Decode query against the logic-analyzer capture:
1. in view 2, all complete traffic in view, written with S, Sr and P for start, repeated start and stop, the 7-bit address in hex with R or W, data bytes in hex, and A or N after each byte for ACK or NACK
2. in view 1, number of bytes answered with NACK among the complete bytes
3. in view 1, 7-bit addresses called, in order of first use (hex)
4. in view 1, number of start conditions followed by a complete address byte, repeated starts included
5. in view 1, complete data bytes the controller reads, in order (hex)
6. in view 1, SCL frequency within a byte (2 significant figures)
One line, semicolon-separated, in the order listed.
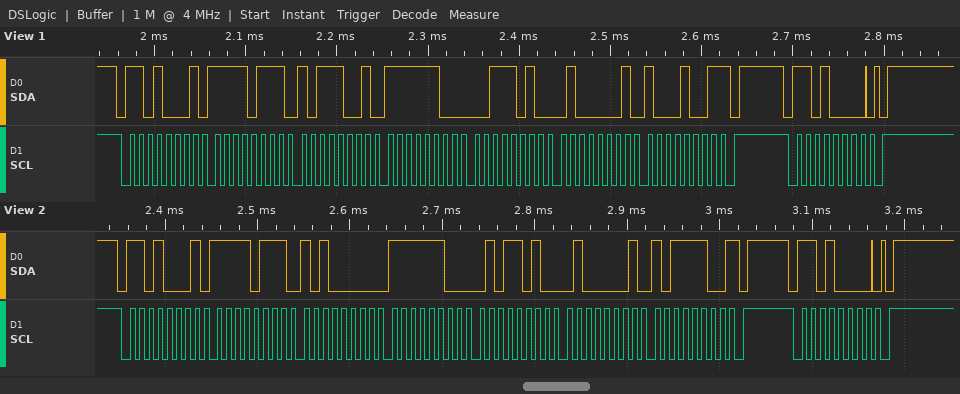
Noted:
S 68R A F7 A A0 A FC A 5A A 41 A BC N P S 68W A P; 1; 0x68; 2; F7 B9 FC 3A 41 89; 100 kHz
